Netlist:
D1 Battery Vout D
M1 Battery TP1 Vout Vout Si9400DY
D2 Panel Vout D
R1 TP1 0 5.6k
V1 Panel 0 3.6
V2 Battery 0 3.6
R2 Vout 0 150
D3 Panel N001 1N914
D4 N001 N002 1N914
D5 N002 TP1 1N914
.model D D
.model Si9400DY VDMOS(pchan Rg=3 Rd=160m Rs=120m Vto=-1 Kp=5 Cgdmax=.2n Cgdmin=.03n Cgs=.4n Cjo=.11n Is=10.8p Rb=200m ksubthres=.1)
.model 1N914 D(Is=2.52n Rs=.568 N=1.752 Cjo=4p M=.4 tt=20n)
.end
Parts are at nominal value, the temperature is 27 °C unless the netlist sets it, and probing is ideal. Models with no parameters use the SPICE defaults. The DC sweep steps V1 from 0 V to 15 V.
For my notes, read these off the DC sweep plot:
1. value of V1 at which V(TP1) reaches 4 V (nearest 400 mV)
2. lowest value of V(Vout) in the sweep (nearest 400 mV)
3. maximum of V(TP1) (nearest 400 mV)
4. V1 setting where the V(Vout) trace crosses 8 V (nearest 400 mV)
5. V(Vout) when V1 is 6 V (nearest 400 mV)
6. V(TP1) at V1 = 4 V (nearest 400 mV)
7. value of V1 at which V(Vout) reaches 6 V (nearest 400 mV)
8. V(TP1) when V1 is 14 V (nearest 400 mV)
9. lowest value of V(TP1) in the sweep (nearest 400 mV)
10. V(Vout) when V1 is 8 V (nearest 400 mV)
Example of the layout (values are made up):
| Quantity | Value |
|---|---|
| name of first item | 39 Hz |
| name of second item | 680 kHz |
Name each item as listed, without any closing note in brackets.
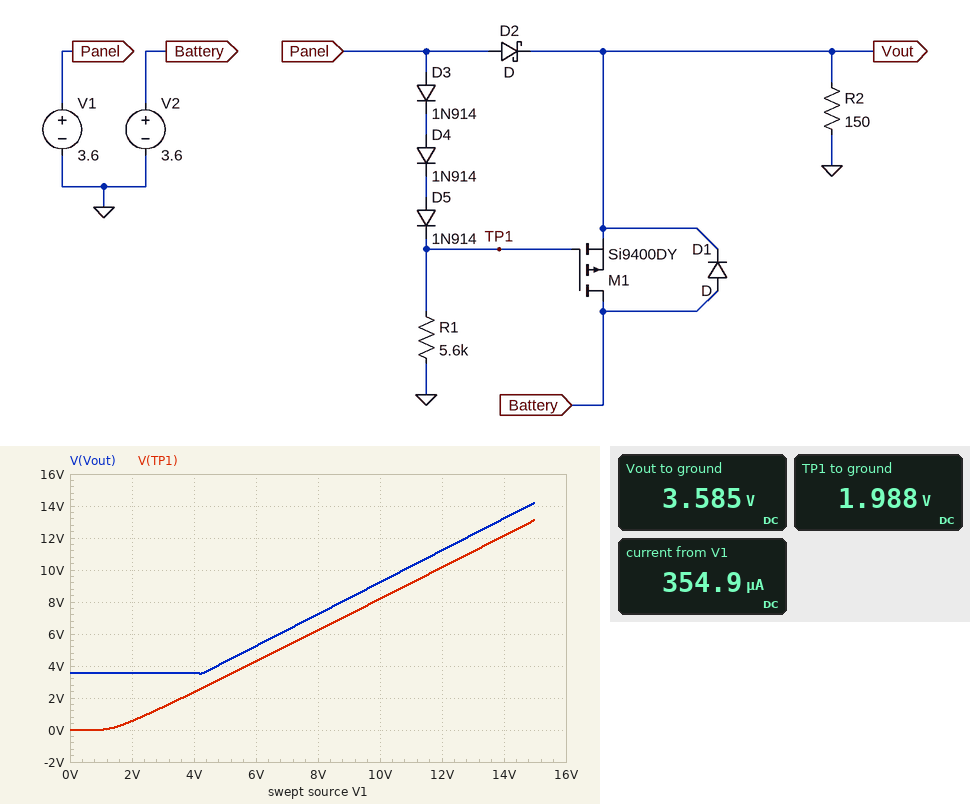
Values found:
| Quantity | Value |
|---|---|
| value of V1 at which V(TP1) reaches 4 V | 5.6 V |
| lowest value of V(Vout) in the sweep | 3.6 V |
| maximum of V(TP1) | 13.2 V |
| V1 setting where the V(Vout) trace crosses 8 V | 8.8 V |
| V(Vout) when V1 is 6 V | 5.2 V |
| V(TP1) at V1 = 4 V | 2.4 V |
| value of V1 at which V(Vout) reaches 6 V | 6.8 V |
| V(TP1) when V1 is 14 V | 12.0 V |
| lowest value of V(TP1) in the sweep | 0 V |
| V(Vout) when V1 is 8 V | 7.2 V |
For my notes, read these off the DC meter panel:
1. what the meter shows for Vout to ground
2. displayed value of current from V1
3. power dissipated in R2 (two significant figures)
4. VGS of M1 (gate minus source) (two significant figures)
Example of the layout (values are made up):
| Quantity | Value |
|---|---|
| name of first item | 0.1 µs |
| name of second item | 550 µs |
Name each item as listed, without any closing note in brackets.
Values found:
| Quantity | Value |
|---|---|
| what the meter shows for Vout to ground | 3.585 V |
| displayed value of current from V1 | 354.9 µA |
| power dissipated in R2 | 86 mW |
| VGS of M1 (gate minus source) | -1.6 V |
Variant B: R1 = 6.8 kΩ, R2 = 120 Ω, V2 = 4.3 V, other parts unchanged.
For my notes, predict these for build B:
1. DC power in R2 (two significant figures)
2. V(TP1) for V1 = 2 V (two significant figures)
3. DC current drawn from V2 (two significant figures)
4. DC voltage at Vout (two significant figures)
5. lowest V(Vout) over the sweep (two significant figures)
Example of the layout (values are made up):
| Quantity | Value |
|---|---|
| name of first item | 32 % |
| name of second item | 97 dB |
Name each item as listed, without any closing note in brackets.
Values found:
| Quantity | Value |
|---|---|
| DC power in R2 | 150 mW |
| V(TP1) for V1 = 2 V | 580 mV |
| DC current drawn from V2 | 36 mA |
| DC voltage at Vout | 4.3 V |
| lowest V(Vout) over the sweep | 4.2 V |
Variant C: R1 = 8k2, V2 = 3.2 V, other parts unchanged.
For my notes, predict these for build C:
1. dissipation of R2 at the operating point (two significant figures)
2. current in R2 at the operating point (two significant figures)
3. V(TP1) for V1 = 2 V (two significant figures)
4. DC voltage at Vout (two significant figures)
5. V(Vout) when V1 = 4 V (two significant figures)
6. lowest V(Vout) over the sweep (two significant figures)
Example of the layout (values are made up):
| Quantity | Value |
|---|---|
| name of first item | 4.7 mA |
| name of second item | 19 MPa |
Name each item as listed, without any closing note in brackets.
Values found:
| Quantity | Value |
|---|---|
| dissipation of R2 at the operating point | 67 mW |
| current in R2 at the operating point | 21 mA |
| V(TP1) for V1 = 2 V | 600 mV |
| DC voltage at Vout | 3.2 V |
| V(Vout) when V1 = 4 V | 3.3 V |
| lowest V(Vout) over the sweep | 3.1 V |
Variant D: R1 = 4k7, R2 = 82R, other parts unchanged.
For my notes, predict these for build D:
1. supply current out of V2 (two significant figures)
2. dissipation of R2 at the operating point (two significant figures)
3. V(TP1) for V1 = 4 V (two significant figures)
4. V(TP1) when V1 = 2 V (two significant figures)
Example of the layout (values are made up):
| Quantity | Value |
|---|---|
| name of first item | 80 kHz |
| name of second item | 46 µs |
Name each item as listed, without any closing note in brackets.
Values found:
| Quantity | Value |
|---|---|
| supply current out of V2 | 44 mA |
| dissipation of R2 at the operating point | 160 mW |
| V(TP1) for V1 = 4 V | 2.3 V |
| V(TP1) when V1 = 2 V | 540 mV |
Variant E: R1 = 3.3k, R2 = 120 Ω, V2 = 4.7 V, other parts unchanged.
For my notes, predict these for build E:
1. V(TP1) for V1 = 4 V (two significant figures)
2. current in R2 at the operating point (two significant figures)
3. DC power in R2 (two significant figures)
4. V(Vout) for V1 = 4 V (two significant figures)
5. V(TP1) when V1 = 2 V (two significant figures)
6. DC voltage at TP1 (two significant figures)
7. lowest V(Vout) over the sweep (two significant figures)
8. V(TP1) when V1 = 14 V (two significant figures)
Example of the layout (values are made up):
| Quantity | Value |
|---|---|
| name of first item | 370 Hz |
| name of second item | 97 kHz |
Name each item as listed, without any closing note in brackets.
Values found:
| Quantity | Value |
|---|---|
| V(TP1) for V1 = 4 V | 2.3 V |
| current in R2 at the operating point | 39 mA |
| DC power in R2 | 180 mW |
| V(Vout) for V1 = 4 V | 4.7 V |
| V(TP1) when V1 = 2 V | 500 mV |
| DC voltage at TP1 | 1.9 V |
| lowest V(Vout) over the sweep | 4.6 V |
| V(TP1) when V1 = 14 V | 12 V |
